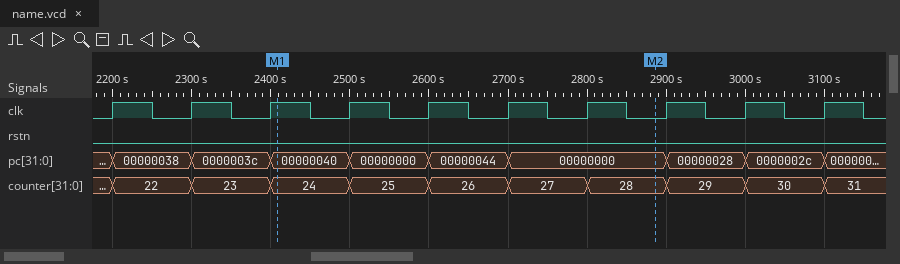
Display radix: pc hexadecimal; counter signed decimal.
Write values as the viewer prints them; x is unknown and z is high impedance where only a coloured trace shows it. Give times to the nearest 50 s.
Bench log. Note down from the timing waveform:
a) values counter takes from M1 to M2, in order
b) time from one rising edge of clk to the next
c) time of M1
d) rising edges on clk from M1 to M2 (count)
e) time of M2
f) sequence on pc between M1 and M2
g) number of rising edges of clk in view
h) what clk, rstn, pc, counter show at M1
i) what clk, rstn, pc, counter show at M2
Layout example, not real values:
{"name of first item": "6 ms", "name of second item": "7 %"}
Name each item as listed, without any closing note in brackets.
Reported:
{"values counter takes from M1 to M2, in order": "24, 25, 26, 27, 28", "time from one rising edge of clk to the next": "100 s", "time of M1": "2400 s", "rising edges on clk from M1 to M2": "4", "time of M2": "2900 s", "sequence on pc between M1 and M2": "00000040, 00000000, 00000044, 00000000", "number of rising edges of clk in view": "10", "what clk, rstn, pc, counter show at M1": "clk=1, rstn=0, pc=00000040, counter=24", "what clk, rstn, pc, counter show at M2": "clk=0, rstn=0, pc=00000000, counter=28"}
